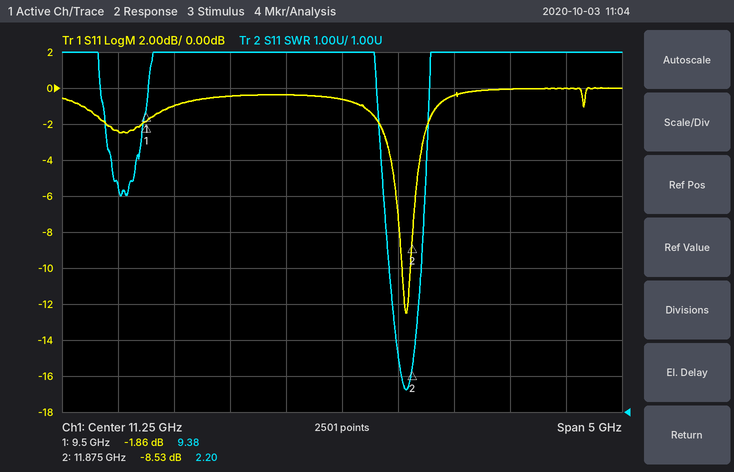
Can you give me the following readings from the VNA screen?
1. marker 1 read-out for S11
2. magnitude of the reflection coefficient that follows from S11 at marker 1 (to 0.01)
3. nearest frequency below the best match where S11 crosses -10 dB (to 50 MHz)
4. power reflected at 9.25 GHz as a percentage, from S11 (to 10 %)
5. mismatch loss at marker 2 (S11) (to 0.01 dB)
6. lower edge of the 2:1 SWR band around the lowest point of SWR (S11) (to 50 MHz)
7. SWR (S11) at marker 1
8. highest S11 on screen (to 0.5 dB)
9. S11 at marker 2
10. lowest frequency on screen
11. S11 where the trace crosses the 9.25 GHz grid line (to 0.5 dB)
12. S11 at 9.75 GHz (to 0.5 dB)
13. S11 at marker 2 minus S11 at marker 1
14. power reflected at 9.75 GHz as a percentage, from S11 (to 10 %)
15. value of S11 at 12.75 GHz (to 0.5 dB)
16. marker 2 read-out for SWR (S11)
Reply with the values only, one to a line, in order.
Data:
-1.86 dB
0.81
11.80 GHz
60 %
0.66 dB
11.80 GHz
9.38
0.0 dB
-8.53 dB
8.75 GHz
-2.5 dB
-1.0 dB
-6.67 dB
80 %
0.0 dB
2.20
